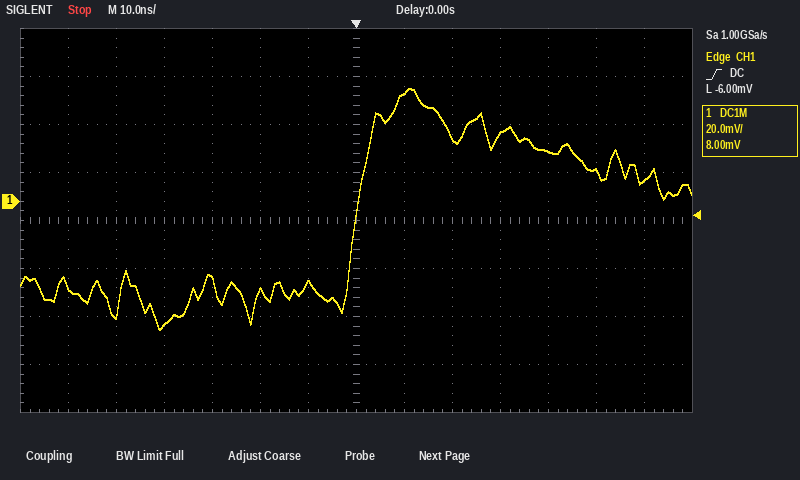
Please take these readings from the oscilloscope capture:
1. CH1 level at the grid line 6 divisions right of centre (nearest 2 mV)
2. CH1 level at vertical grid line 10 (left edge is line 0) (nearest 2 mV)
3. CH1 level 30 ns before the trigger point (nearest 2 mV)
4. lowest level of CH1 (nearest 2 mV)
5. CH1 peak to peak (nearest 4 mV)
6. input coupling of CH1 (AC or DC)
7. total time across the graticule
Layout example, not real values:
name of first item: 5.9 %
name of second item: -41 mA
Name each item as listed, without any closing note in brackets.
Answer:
CH1 level at the grid line 6 divisions right of centre: 8 mV
CH1 level at vertical grid line 10 (left edge is line 0): 28 mV
CH1 level 30 ns before the trigger point: -32 mV
lowest level of CH1: -54 mV
CH1 peak to peak: 100 mV
input coupling of CH1: DC
total time across the graticule: 140 ns
